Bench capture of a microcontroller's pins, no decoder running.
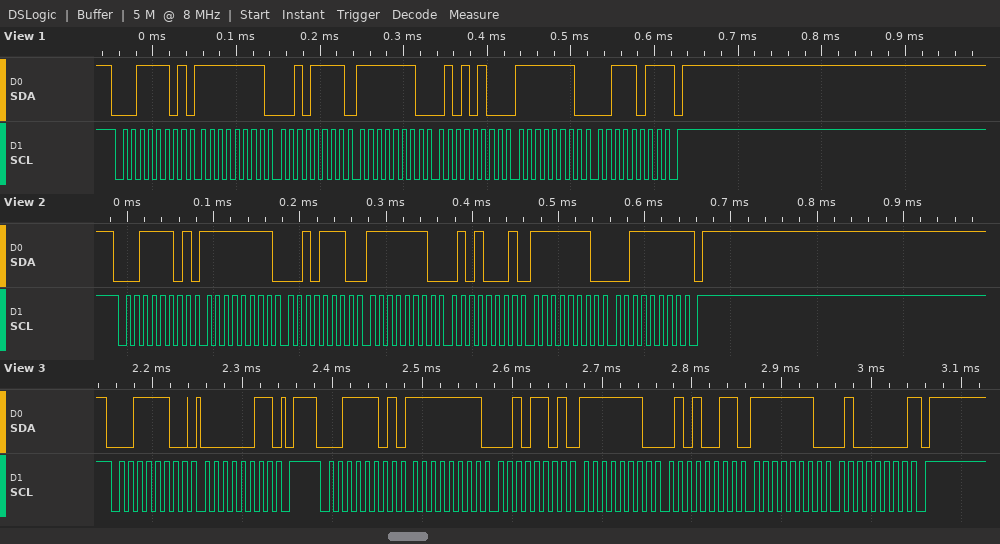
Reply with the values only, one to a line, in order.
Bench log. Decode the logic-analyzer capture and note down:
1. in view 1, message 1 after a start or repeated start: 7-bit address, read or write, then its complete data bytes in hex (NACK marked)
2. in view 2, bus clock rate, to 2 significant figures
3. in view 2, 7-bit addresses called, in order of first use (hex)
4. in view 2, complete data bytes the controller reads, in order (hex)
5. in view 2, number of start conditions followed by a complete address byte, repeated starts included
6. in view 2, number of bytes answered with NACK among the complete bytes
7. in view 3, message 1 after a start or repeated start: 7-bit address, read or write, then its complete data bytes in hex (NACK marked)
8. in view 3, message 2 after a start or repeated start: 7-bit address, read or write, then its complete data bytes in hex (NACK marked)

0x1E read: FF 2F FE 54 FE 3B NACK
100 kHz
0x1E
FF 2E FE 51 FE 3F
1
1
0x1E write: 03
0x1E read: FF 2D FE 53 FE 40 NACK
